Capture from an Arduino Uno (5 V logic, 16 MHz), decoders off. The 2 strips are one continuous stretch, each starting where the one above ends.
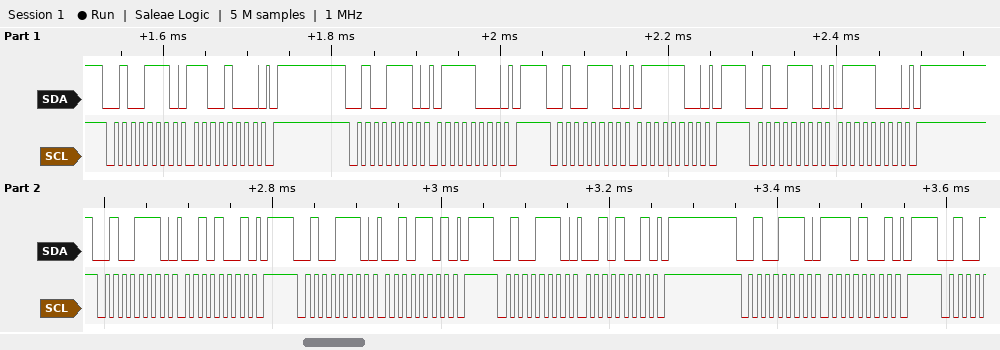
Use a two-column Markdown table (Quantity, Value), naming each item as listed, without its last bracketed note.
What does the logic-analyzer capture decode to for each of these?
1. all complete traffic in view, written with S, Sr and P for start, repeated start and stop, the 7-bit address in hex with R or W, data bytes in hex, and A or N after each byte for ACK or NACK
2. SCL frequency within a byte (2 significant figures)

| Quantity | Value |
|---|---|
| all complete traffic in view, written with S, Sr and P for start, repeated start and stop, the 7-bit address in hex with R or W, data bytes in hex, and A or N after each byte for ACK or NACK | S 27W A C8 A P S 27W A 78 A P S 27W A 7C A P S 27W A 78 A P S 27W A 29 A P S 27W A 2D A P S 27W A 29 A P S 27W A E9 A P |
| SCL frequency within a byte | 100 kHz |
